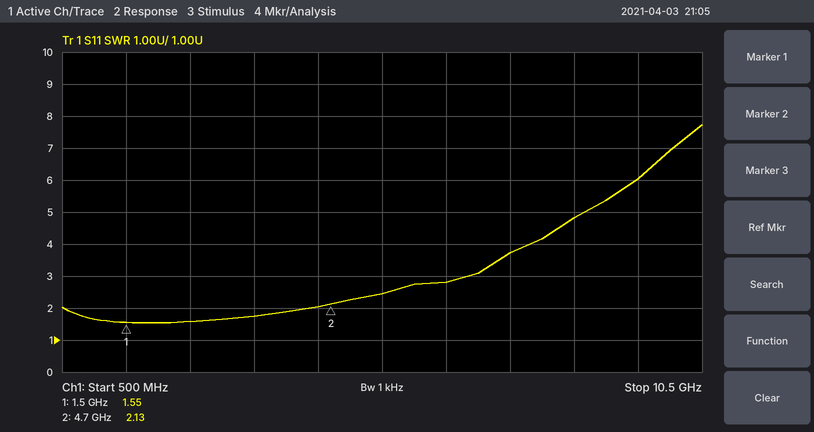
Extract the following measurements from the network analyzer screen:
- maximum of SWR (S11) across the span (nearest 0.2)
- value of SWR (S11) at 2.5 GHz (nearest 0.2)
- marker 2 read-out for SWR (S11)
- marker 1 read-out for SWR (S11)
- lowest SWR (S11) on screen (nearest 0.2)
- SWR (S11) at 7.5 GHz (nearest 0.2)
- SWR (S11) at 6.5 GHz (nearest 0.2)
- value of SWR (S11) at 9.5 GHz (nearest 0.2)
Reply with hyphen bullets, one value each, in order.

- 7.8
- 1.6
- 2.13
- 1.55
- 1.6
- 3.8
- 2.8
- 6.0
